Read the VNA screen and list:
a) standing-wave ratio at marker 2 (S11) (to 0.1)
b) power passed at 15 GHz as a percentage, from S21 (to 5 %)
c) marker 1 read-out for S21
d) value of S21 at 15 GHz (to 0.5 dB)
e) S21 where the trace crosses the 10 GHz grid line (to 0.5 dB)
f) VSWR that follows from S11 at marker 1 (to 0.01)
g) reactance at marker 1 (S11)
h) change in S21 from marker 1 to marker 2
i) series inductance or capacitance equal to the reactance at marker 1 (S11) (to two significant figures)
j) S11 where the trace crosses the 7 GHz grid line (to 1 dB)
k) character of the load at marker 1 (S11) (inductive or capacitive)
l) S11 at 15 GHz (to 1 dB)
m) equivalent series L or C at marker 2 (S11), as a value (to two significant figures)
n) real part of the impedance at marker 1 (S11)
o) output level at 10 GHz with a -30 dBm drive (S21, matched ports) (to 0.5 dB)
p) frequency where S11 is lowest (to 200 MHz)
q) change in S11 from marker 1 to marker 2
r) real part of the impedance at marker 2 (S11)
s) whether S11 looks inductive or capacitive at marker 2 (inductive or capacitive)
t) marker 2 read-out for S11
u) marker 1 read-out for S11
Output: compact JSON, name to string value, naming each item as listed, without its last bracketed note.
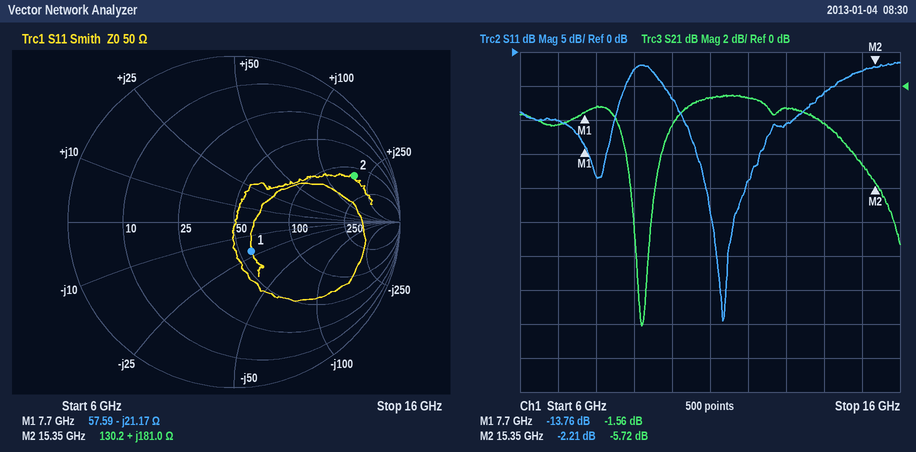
{"standing-wave ratio at marker 2 (S11)": "7.9", "power passed at 15 GHz as a percentage, from S21": "35 %", "marker 1 read-out for S21": "-1.56 dB", "value of S21 at 15 GHz": "-4.5 dB", "S21 where the trace crosses the 10 GHz grid line": "-2.5 dB", "VSWR that follows from S11 at marker 1": "1.52", "reactance at marker 1": "-21.17 Ω", "change in S21 from marker 1 to marker 2": "-4.16 dB", "series inductance or capacitance equal to the reactance at marker 1 (S11)": "980 fF", "S11 where the trace crosses the 7 GHz grid line": "-10 dB", "character of the load at marker 1 (S11)": "capacitive", "S11 at 15 GHz": "-3 dB", "equivalent series L or C at marker 2 (S11), as a value": "1.9 nH", "real part of the impedance at marker 1": "57.59 Ω", "output level at 10 GHz with a -30 dBm drive (S21, matched ports)": "-32.5 dBm", "frequency where S11 is lowest": "11.4 GHz", "change in S11 from marker 1 to marker 2": "11.55 dB", "real part of the impedance at marker 2": "130.2 Ω", "whether S11 looks inductive or capacitive at marker 2": "inductive", "marker 2 read-out for S11": "-2.21 dB", "marker 1 read-out for S11": "-13.76 dB"}
